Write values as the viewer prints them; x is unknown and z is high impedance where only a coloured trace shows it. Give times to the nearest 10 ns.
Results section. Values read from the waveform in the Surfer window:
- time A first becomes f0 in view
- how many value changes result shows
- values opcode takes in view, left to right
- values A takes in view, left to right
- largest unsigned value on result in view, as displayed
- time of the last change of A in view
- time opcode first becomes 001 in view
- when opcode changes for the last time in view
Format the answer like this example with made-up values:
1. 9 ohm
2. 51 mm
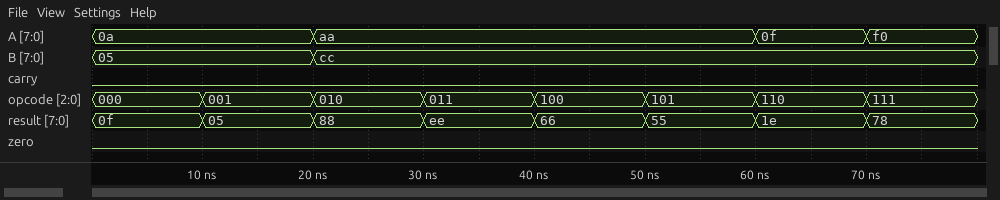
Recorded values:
1. 70 ns
2. 7
3. 000, 001, 010, 011, 100, 101, 110, 111
4. 0a, aa, 0f, f0
5. ee
6. 70 ns
7. 10 ns
8. 70 ns
